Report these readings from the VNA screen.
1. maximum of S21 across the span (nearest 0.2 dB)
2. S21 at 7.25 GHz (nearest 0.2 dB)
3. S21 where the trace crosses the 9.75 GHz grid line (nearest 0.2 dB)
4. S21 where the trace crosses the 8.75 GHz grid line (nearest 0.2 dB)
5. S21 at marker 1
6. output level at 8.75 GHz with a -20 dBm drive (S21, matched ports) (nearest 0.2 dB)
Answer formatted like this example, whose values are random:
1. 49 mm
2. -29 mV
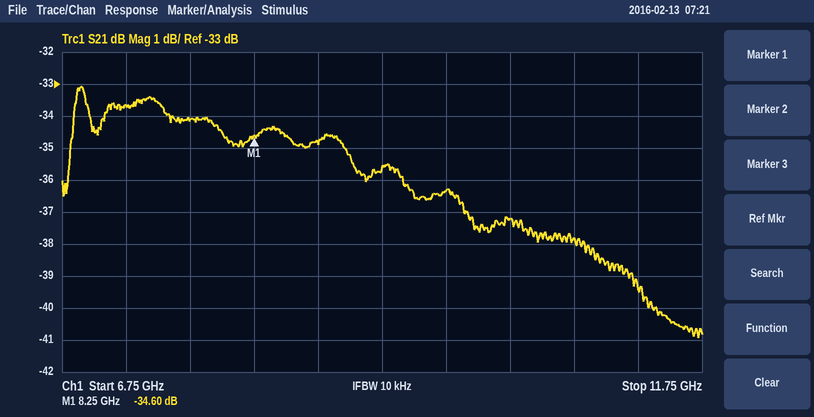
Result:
1. -33.0 dB
2. -33.6 dB
3. -36.4 dB
4. -34.8 dB
5. -34.60 dB
6. -54.8 dBm
